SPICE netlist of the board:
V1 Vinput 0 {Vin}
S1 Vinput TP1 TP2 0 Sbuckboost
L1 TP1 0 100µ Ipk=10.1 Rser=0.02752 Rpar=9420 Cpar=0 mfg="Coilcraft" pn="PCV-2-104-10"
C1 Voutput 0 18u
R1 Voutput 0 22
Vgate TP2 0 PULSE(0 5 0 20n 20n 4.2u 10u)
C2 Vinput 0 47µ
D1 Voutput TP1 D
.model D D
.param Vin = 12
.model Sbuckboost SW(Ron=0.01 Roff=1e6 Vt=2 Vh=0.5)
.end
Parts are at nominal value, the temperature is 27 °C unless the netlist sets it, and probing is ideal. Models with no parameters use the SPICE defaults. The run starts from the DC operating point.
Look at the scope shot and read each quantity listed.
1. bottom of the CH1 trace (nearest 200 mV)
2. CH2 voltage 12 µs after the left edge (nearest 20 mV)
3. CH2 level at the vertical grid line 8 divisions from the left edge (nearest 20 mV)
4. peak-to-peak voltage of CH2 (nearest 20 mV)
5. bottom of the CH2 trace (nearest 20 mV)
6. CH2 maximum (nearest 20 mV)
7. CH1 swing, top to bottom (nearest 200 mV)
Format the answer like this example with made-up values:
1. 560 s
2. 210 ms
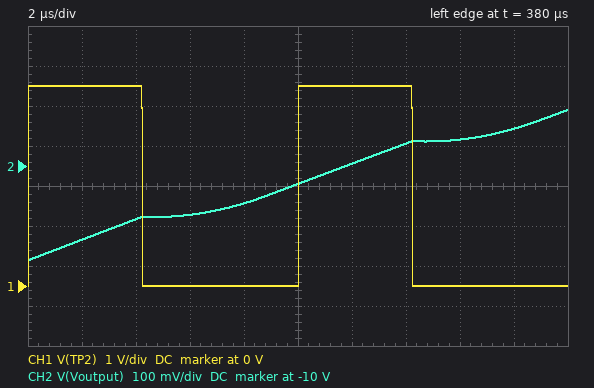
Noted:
1. 0 V
2. -10.00 V
3. -9.94 V
4. 380 mV
5. -10.24 V
6. -9.86 V
7. 5.0 V
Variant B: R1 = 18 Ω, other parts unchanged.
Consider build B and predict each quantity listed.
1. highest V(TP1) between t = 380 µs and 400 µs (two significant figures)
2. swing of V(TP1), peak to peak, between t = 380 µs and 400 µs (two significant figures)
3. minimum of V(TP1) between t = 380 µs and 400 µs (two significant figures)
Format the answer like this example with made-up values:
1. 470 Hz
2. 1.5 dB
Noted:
1. 12 V
2. 22 V
3. -10 V
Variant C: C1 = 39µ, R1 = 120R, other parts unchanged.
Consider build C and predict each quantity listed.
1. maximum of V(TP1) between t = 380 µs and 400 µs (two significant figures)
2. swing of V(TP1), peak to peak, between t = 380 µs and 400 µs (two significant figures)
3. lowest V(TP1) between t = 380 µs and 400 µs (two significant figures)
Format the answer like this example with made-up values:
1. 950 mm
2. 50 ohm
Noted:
1. 12 V
2. 28 V
3. -16 V
